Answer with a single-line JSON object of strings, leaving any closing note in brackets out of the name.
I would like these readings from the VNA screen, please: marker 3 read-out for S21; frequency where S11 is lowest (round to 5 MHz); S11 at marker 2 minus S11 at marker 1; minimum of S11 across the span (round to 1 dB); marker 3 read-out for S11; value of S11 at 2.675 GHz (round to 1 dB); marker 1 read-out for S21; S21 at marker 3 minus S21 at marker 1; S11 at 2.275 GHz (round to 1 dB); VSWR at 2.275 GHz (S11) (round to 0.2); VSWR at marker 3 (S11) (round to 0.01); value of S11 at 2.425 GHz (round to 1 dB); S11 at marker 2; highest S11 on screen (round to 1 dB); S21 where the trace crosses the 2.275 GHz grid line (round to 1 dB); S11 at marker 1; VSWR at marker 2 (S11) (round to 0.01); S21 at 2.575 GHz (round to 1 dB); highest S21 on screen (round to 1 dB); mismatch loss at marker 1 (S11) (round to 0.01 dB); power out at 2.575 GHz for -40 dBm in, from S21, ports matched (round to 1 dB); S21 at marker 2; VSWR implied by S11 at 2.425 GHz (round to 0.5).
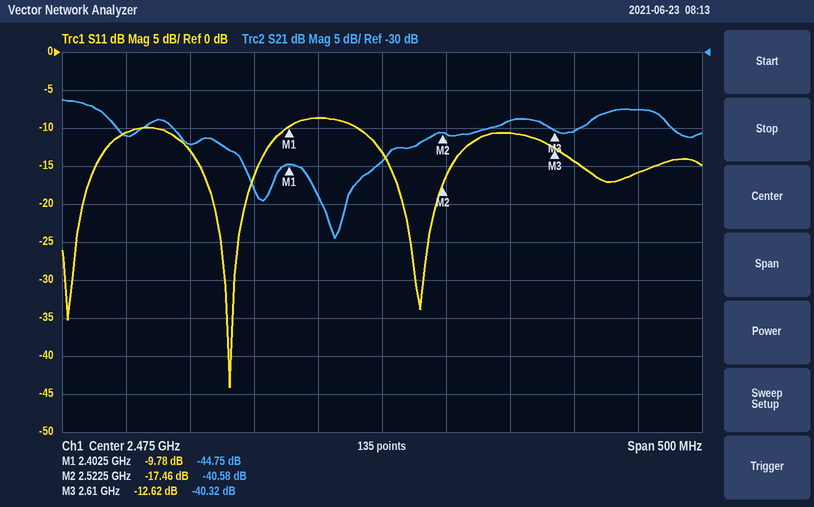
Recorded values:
{"marker 3 read-out for S21": "-40.32 dB", "frequency where S11 is lowest": "2.355 GHz", "S11 at marker 2 minus S11 at marker 1": "-7.68 dB", "minimum of S11 across the span": "-44 dB", "marker 3 read-out for S11": "-12.62 dB", "value of S11 at 2.675 GHz": "-16 dB", "marker 1 read-out for S21": "-44.75 dB", "S21 at marker 3 minus S21 at marker 1": "4.43 dB", "S11 at 2.275 GHz": "-11 dB", "VSWR at 2.275 GHz (S11)": "1.8", "VSWR at marker 3 (S11)": "1.61", "value of S11 at 2.425 GHz": "-9 dB", "S11 at marker 2": "-17.46 dB", "highest S11 on screen": "-9 dB", "S21 where the trace crosses the 2.275 GHz grid line": "-41 dB", "S11 at marker 1": "-9.78 dB", "VSWR at marker 2 (S11)": "1.31", "S21 at 2.575 GHz": "-39 dB", "highest S21 on screen": "-36 dB", "mismatch loss at marker 1 (S11)": "0.48 dB", "power out at 2.575 GHz for -40 dBm in, from S21, ports matched": "-79 dBm", "S21 at marker 2": "-40.58 dB", "VSWR implied by S11 at 2.425 GHz": "2.0"}
